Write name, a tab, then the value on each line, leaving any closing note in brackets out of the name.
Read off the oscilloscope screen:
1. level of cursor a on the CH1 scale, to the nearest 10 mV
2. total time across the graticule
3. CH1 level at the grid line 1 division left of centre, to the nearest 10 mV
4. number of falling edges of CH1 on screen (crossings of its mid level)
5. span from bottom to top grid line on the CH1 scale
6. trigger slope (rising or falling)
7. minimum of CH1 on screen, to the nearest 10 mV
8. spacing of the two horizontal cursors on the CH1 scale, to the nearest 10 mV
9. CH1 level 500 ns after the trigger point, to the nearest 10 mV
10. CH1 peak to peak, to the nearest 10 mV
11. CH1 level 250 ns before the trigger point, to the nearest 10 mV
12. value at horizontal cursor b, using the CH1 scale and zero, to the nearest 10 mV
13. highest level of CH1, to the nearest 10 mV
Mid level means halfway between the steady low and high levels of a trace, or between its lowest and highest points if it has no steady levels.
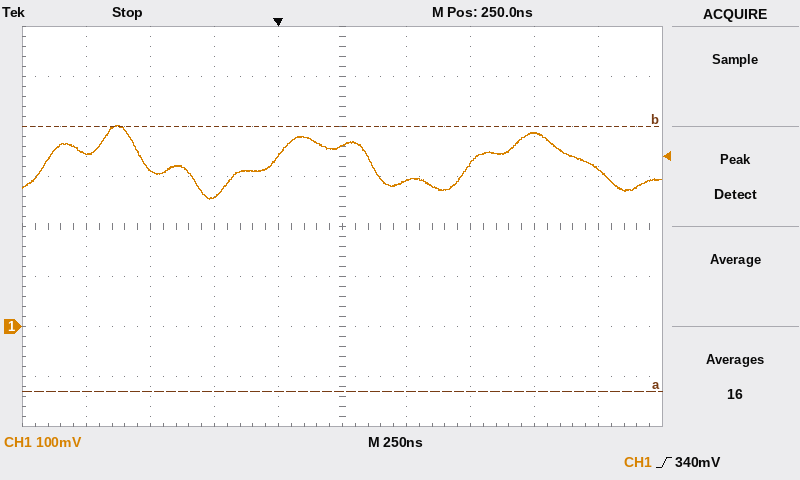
level of cursor a on the CH1 scale, to the nearest 10 mV	-130 mV
total time across the graticule	2.5 µs
CH1 level at the grid line 1 division left of centre, to the nearest 10 mV	340 mV
number of falling edges of CH1 on screen	3
span from bottom to top grid line on the CH1 scale	800 mV
trigger slope	rising
minimum of CH1 on screen, to the nearest 10 mV	250 mV
spacing of the two horizontal cursors on the CH1 scale, to the nearest 10 mV	530 mV
CH1 level 500 ns after the trigger point, to the nearest 10 mV	290 mV
CH1 peak to peak, to the nearest 10 mV	150 mV
CH1 level 250 ns before the trigger point, to the nearest 10 mV	260 mV
value at horizontal cursor b, using the CH1 scale and zero, to the nearest 10 mV	400 mV
highest level of CH1, to the nearest 10 mV	400 mV
